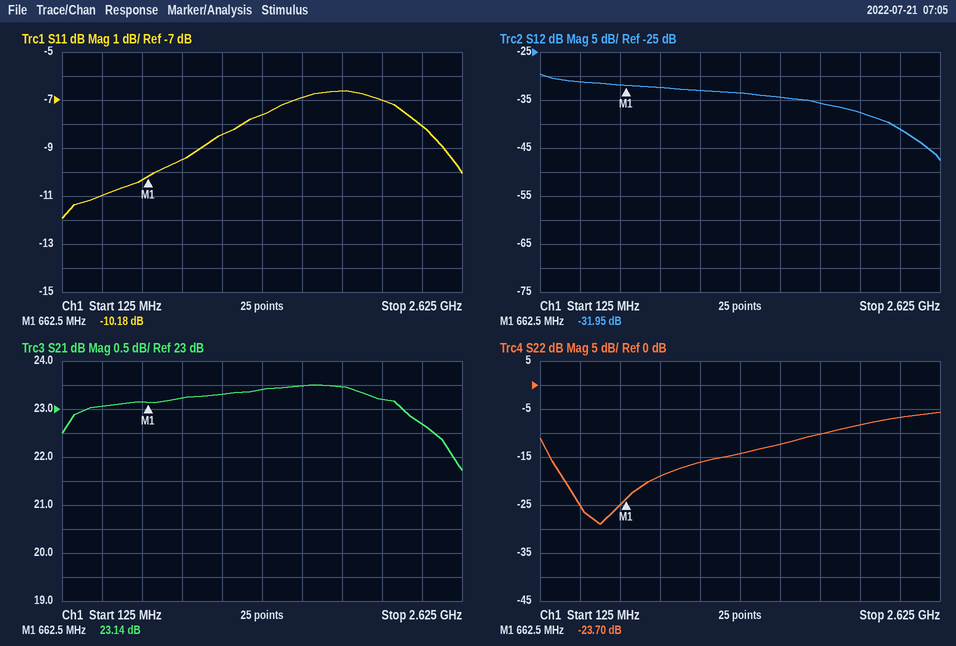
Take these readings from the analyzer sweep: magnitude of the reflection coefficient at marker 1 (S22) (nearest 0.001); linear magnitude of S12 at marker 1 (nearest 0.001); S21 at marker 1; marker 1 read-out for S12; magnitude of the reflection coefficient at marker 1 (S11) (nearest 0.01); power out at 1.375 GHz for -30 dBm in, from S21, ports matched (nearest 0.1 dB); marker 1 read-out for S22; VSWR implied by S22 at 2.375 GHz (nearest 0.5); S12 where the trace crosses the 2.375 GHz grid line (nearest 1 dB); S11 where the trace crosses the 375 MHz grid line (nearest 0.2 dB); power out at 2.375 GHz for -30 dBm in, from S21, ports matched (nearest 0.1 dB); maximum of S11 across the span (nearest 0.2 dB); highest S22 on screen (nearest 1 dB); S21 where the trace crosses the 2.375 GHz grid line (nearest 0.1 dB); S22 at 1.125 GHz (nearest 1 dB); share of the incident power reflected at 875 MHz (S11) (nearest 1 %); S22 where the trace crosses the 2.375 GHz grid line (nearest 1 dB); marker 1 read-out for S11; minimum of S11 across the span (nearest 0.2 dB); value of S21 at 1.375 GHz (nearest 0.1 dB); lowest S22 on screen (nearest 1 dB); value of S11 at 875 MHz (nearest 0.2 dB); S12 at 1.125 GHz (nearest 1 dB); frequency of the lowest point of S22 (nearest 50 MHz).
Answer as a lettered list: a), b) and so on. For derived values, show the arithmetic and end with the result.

a) 10^(-23.7/20) ≈ 0.065
b) 10^(-31.95/20) ≈ 0.025
c) 23.14 dB
d) -31.95 dB
e) 10^(-10.18/20) ≈ 0.31
f) -30 dBm + (23.4 dB) = -6.6 dBm
g) -23.70 dB
h) |Γ| = 10^(-7/20) = 0.4467; VSWR = (1 + 0.4467)/(1 − 0.4467) ≈ 2.61, so 2.5 to the nearest 0.5
i) -41 dB
j) -11.0 dB
k) -30 dBm + (22.7 dB) = -7.3 dBm
l) -6.6 dB
m) -6 dB
n) 22.7 dB
o) -16 dB
p) 10^(-9.4/10) ≈ 11 %
q) -7 dB
r) -10.18 dB
s) -12.0 dB
t) 23.4 dB
u) -29 dB
v) -9.4 dB
w) -33 dB
x) 500 MHz
